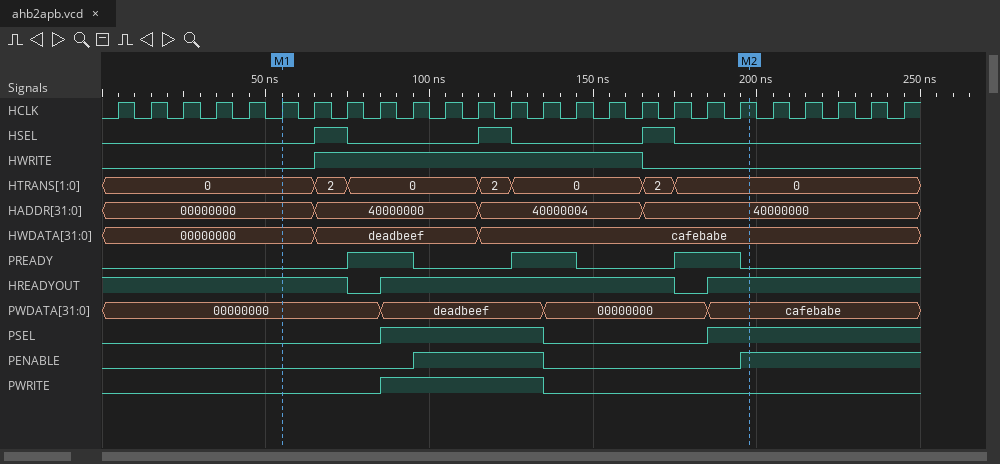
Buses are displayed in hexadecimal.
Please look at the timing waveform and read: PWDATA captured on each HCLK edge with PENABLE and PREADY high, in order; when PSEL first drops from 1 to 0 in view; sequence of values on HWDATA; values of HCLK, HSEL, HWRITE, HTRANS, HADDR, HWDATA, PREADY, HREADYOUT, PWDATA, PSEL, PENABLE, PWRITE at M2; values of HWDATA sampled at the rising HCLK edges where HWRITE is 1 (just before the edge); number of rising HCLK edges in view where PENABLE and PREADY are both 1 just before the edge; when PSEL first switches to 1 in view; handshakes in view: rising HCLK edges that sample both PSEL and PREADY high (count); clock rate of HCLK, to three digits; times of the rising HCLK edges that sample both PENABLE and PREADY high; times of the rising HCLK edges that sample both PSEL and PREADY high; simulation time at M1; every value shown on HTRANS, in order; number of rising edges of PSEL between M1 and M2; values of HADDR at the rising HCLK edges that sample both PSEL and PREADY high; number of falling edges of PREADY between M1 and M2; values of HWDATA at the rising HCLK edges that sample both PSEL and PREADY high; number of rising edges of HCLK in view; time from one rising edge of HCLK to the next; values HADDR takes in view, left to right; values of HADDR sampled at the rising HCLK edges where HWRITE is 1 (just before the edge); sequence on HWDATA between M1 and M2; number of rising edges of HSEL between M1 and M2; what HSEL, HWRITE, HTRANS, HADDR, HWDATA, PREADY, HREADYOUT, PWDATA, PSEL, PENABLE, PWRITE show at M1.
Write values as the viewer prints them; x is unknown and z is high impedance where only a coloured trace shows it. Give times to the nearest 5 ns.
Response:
deadbeef
135 ns
00000000, deadbeef, cafebabe
HCLK=1, HSEL=0, HWRITE=0, HTRANS=0, HADDR=40000000, HWDATA=cafebabe, PREADY=0, HREADYOUT=1, PWDATA=cafebabe, PSEL=1, PENABLE=1, PWRITE=0
deadbeef, deadbeef, deadbeef, deadbeef, deadbeef, cafebabe, cafebabe, cafebabe, cafebabe, cafebabe
1
85 ns
3
100 MHz
135 ns
95 ns, 135 ns, 195 ns
55 ns
0, 2, 0, 2, 0, 2, 0
2
40000000, 40000004, 40000000
3
deadbeef, cafebabe, cafebabe
25
10 ns
00000000, 40000000, 40000004, 40000000
40000000, 40000000, 40000000, 40000000, 40000000, 40000004, 40000004, 40000004, 40000004, 40000004
00000000, deadbeef, cafebabe
3
HSEL=0, HWRITE=0, HTRANS=0, HADDR=00000000, HWDATA=00000000, PREADY=0, HREADYOUT=1, PWDATA=00000000, PSEL=0, PENABLE=0, PWRITE=0
